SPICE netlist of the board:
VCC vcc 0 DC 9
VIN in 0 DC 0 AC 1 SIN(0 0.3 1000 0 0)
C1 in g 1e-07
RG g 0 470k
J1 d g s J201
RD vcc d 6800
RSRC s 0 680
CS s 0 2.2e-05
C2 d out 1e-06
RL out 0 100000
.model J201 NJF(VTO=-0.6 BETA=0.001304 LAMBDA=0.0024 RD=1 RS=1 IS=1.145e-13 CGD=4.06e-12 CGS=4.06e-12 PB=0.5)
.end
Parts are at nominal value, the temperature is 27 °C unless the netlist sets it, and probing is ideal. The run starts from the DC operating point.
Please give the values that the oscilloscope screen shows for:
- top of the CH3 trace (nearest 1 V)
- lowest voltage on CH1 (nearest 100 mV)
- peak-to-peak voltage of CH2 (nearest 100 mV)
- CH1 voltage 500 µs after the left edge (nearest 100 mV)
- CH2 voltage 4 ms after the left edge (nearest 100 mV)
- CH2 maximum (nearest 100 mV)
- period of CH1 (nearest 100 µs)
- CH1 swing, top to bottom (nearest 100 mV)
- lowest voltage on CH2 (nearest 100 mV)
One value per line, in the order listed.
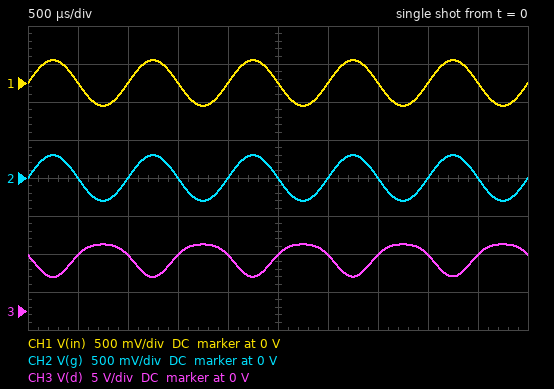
9 V
-300 mV
600 mV
0 V
0 V
300 mV
1.0 ms
600 mV
-300 mV
